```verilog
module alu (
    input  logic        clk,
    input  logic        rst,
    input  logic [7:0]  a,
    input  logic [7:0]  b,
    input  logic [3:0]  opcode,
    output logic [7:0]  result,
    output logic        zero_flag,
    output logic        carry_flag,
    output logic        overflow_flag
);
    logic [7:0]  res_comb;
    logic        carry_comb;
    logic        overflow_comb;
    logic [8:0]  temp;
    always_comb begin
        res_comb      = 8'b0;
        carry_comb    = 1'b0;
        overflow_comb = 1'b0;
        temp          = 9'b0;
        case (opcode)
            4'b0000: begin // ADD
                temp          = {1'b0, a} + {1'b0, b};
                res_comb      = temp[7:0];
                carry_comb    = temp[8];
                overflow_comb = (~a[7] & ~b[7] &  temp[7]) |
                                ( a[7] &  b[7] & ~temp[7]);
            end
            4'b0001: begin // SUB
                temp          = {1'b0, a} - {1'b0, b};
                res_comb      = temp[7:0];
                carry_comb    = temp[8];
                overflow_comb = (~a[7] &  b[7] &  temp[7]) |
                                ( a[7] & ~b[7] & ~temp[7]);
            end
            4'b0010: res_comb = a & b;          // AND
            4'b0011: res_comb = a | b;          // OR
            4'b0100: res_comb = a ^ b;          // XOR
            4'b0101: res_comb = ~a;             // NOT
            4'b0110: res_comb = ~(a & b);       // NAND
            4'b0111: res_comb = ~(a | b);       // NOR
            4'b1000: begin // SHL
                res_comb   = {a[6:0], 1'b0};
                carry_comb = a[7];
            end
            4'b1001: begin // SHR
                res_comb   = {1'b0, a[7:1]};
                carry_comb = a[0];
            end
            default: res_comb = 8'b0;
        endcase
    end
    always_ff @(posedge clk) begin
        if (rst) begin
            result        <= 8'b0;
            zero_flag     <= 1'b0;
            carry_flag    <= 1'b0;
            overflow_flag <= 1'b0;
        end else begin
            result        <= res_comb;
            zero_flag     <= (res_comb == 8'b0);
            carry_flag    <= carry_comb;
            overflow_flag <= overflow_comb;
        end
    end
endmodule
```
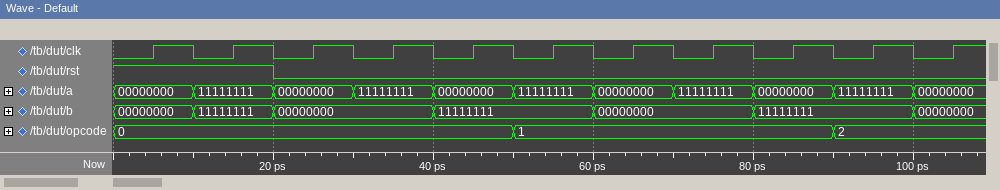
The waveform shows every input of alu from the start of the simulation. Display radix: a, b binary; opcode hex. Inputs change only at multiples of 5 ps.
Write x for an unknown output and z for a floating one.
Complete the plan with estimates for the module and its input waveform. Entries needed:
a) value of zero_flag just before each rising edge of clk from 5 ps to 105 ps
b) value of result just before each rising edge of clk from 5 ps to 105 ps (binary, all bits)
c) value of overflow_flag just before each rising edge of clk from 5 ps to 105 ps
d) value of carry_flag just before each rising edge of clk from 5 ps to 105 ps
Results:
x 0 0 1 0 0 1 1 0 0 0
x, 00000000, 00000000, 00000000, 11111111, 11111111, 00000000, 00000000, 11111111, 00000001, 11111111
x 0 0 0 0 0 0 0 0 0 0
x 0 0 0 0 0 0 0 0 1 0
